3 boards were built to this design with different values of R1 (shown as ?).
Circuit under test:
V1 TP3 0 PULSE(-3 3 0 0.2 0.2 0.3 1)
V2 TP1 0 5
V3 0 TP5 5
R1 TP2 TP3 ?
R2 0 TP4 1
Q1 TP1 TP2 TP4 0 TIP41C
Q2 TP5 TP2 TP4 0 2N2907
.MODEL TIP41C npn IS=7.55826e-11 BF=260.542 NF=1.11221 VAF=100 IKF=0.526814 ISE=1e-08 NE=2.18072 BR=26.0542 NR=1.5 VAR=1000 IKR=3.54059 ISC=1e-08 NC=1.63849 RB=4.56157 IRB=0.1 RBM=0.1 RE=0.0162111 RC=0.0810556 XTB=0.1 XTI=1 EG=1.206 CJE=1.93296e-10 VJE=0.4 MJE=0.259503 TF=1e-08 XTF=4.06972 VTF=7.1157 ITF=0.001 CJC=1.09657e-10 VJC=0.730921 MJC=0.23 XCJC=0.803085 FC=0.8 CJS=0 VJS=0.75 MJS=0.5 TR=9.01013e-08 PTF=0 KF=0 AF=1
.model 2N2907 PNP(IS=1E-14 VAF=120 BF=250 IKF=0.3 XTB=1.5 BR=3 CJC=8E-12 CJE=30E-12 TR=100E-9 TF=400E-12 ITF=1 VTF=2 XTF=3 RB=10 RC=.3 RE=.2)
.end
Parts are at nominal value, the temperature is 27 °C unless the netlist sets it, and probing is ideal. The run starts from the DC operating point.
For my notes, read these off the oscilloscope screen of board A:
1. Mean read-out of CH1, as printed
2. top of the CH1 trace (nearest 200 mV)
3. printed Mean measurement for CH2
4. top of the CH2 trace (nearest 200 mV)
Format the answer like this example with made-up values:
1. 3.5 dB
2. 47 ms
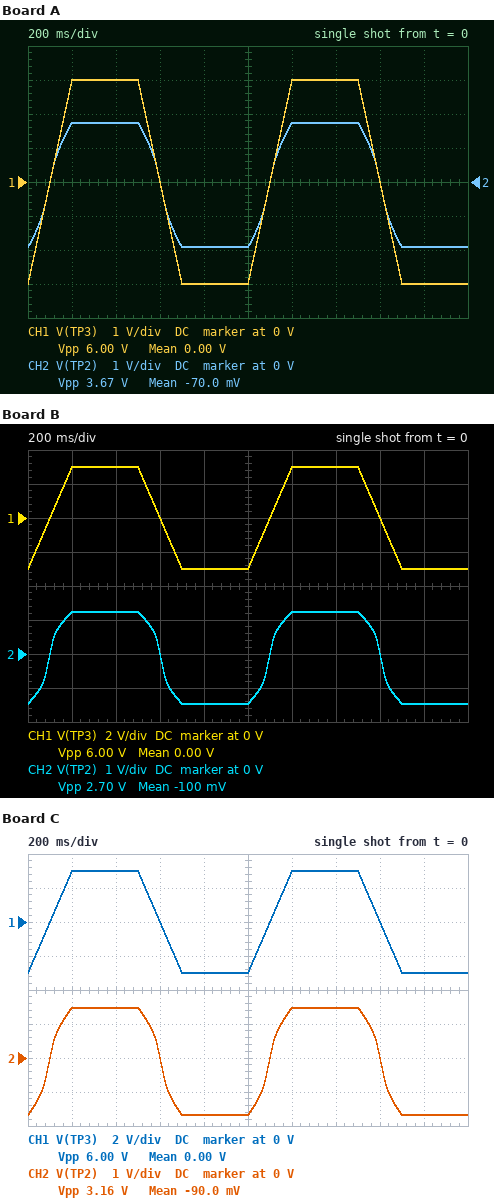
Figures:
1. 0.00 V
2. 3.0 V
3. -70.0 mV
4. 1.8 V
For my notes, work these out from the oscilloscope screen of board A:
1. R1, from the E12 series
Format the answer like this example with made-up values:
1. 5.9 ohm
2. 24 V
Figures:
1. 100 Ω
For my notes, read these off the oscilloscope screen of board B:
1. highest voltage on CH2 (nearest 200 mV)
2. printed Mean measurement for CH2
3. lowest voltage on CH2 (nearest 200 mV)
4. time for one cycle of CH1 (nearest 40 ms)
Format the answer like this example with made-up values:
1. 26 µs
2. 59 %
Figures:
1. 1.2 V
2. -100 mV
3. -1.4 V
4. 1.00 s
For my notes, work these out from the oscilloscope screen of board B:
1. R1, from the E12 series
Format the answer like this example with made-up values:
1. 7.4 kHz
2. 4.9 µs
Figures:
1. 330 Ω
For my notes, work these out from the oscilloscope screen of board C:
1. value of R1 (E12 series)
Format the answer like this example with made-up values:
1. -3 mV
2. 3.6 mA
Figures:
1. 180 Ω
